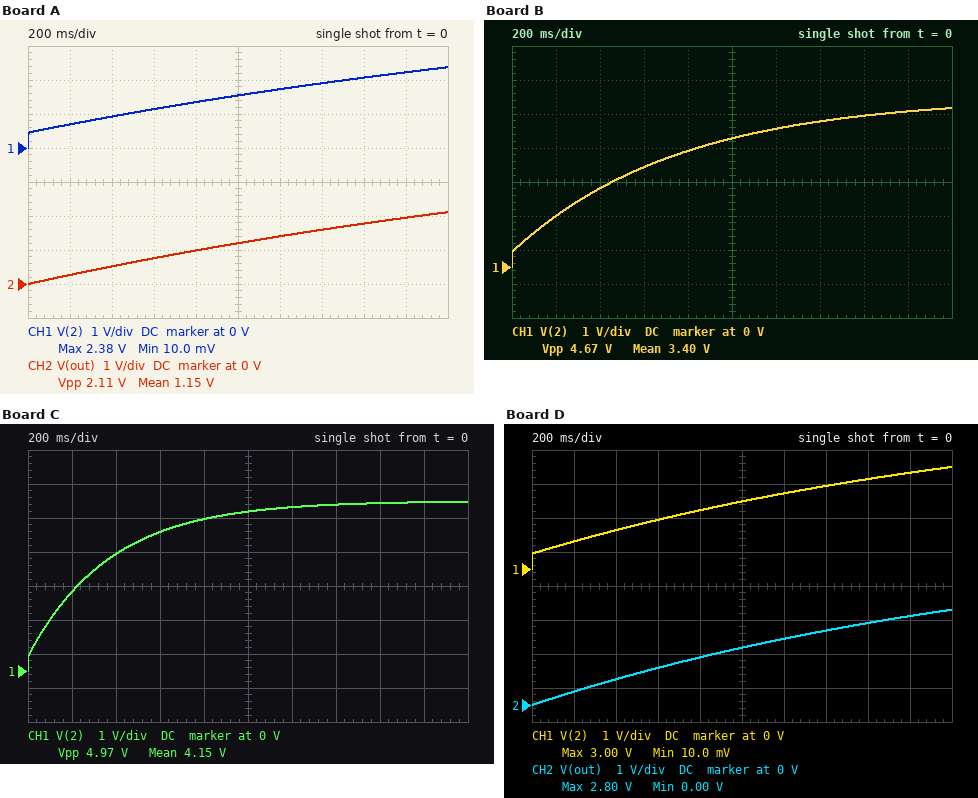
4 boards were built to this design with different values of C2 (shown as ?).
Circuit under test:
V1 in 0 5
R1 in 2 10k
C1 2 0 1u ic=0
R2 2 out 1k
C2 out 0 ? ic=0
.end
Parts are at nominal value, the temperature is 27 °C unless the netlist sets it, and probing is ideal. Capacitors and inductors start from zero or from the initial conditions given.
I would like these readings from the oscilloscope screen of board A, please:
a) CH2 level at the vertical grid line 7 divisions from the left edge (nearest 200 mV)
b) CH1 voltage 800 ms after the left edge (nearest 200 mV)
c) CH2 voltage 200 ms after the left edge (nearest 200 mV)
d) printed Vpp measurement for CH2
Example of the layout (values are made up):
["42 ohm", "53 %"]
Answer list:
["1.6 V", "1.4 V", "200 mV", "2.11 V"]
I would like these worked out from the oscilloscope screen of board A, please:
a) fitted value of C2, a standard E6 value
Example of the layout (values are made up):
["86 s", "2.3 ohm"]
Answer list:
["330 µF"]
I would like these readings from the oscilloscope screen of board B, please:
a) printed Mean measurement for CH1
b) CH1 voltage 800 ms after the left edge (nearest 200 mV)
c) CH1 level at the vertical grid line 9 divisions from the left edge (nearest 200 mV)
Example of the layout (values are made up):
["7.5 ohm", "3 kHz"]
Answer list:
["3.40 V", "3.4 V", "4.6 V"]
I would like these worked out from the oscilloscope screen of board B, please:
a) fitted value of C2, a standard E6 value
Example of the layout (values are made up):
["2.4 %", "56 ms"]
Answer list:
["68 µF"]
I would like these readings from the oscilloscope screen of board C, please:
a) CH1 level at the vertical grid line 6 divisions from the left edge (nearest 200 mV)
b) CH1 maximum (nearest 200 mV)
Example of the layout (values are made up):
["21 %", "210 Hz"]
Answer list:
["4.8 V", "5.0 V"]
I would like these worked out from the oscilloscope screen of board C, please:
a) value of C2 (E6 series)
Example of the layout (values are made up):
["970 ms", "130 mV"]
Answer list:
["33 µF"]
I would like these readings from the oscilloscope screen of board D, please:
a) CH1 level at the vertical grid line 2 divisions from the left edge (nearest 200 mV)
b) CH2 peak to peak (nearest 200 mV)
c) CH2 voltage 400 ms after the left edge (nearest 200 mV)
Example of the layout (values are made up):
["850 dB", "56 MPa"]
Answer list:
["1.2 V", "2.8 V", "800 mV"]
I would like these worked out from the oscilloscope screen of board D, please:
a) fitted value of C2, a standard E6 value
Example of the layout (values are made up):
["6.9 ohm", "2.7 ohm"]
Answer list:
["220 µF"]
